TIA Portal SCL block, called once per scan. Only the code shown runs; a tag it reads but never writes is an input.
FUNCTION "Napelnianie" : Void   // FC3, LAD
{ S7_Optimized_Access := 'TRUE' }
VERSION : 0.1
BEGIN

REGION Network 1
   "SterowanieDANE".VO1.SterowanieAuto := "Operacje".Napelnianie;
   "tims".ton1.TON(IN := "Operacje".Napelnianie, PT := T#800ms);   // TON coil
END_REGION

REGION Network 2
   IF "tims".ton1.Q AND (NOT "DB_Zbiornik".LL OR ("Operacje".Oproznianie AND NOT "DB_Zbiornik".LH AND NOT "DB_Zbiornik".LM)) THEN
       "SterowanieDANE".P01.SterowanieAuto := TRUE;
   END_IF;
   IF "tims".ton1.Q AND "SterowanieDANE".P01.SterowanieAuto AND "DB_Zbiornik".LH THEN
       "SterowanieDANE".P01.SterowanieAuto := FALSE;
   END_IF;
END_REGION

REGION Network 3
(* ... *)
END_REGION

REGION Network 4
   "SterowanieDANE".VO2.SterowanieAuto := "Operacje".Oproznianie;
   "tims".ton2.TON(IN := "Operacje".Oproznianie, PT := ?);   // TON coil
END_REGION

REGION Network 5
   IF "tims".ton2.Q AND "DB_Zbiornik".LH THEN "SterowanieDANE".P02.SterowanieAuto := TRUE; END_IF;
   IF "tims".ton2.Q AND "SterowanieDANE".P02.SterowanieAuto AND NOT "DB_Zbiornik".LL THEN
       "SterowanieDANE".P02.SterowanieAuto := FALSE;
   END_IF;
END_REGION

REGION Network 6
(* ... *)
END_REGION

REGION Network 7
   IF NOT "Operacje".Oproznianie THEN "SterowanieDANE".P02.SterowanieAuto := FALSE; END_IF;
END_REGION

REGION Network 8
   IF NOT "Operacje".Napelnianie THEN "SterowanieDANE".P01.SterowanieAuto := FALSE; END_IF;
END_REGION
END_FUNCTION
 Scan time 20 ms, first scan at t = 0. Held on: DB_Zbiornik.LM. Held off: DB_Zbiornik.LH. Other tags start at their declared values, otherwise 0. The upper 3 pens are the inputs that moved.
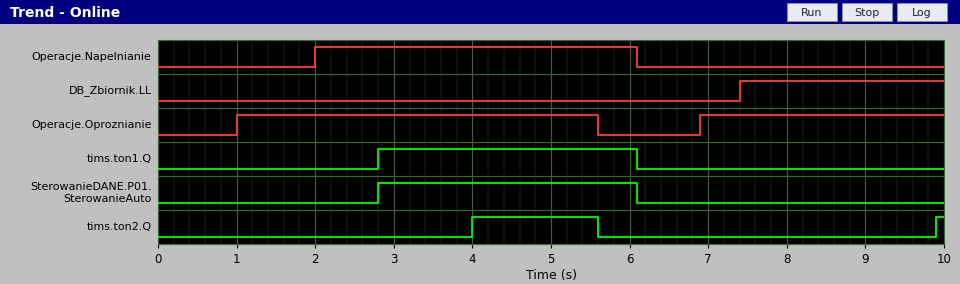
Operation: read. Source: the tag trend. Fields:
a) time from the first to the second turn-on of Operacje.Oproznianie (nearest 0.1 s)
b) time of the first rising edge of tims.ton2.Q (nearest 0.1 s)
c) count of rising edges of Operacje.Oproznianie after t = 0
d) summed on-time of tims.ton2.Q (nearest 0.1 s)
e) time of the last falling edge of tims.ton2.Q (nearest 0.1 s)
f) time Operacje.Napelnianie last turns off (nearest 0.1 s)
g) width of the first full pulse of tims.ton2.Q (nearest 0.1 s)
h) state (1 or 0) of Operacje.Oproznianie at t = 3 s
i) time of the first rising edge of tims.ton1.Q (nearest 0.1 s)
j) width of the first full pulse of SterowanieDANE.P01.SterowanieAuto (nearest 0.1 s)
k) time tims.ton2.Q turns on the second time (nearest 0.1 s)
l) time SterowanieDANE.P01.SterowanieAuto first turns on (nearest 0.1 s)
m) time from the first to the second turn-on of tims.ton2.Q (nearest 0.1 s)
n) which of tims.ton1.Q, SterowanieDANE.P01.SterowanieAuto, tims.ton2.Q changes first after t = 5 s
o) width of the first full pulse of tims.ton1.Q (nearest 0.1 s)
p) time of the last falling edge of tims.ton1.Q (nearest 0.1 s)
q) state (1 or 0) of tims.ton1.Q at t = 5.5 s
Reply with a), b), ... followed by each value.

a) 5.9 s
b) 4.0 s
c) 2
d) 1.7 s
e) 5.6 s
f) 6.1 s
g) 1.6 s
h) 1
i) 2.8 s
j) 3.3 s
k) 9.9 s
l) 2.8 s
m) 5.9 s
n) tims.ton2.Q
o) 3.3 s
p) 6.1 s
q) 1
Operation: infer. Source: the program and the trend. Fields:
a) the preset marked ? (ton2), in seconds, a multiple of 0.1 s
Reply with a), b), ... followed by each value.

a) 3.0 s
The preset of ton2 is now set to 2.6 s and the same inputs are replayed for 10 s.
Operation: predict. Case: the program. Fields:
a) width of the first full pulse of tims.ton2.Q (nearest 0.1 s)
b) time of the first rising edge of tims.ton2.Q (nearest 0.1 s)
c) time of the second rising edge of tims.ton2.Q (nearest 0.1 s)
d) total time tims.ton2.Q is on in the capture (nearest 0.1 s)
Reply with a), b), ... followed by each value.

a) 2.0 s
b) 3.6 s
c) 9.5 s
d) 2.5 s
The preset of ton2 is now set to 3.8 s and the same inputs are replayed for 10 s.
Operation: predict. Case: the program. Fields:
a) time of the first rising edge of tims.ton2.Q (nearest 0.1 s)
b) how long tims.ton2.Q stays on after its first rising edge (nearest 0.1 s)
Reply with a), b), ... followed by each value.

a) 4.8 s
b) 0.8 s
